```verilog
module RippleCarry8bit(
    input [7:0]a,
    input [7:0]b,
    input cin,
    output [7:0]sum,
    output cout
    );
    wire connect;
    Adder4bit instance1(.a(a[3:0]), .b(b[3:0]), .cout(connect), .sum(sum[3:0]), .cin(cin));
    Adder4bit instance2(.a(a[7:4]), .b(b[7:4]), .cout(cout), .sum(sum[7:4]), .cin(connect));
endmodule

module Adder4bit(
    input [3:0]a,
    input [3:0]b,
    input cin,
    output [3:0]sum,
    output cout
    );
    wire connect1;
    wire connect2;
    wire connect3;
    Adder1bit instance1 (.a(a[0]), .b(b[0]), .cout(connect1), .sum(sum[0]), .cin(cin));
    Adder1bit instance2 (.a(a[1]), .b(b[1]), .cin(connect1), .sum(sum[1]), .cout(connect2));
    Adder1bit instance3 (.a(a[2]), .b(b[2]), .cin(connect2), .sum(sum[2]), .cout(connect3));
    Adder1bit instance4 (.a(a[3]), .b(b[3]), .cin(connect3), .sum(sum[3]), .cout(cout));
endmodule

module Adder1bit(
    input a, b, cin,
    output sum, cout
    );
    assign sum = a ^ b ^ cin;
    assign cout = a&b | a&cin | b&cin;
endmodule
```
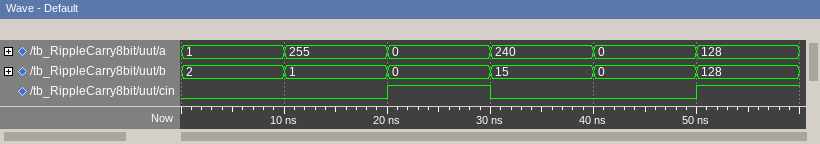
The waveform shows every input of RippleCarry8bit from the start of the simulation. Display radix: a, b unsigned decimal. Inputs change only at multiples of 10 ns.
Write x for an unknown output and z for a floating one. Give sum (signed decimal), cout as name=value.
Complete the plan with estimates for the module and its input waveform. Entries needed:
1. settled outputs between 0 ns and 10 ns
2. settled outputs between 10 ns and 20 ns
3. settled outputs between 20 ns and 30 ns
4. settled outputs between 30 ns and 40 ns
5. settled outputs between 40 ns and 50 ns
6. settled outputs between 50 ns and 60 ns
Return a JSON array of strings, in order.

["sum=3, cout=0", "sum=0, cout=1", "sum=1, cout=0", "sum=-1, cout=0", "sum=0, cout=0", "sum=1, cout=1"]
